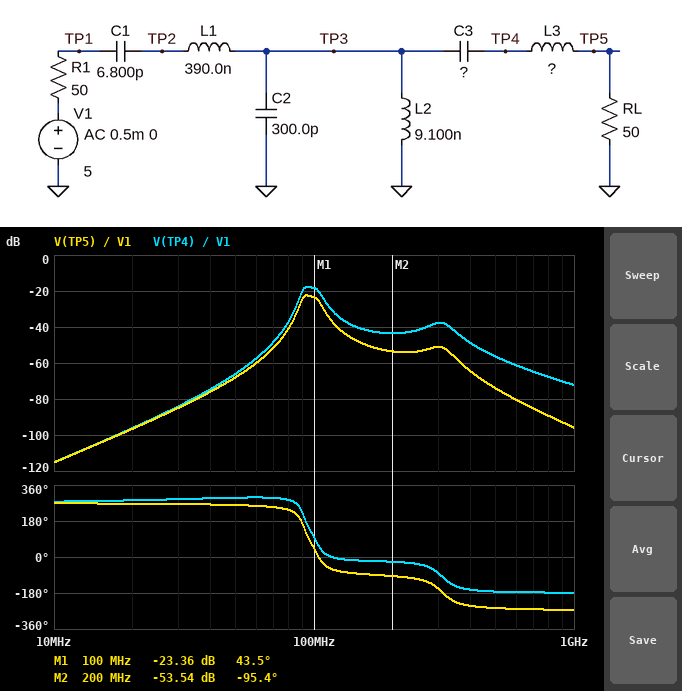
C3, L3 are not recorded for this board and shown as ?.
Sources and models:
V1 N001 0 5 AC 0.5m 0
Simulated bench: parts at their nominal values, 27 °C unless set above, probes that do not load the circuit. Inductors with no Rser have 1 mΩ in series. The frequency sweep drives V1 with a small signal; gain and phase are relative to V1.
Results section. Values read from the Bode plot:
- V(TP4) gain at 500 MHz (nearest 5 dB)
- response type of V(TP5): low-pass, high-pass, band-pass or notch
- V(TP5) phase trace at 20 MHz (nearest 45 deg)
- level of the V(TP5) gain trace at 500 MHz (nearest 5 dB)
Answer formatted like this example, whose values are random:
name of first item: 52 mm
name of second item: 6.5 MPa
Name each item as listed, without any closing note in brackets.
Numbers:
V(TP4) gain at 500 MHz: -55 dB
response type of V(TP5): low-pass, high-pass, band-pass or notch: band-pass
V(TP5) phase trace at 20 MHz: 270 deg
level of the V(TP5) gain trace at 500 MHz: -75 dB
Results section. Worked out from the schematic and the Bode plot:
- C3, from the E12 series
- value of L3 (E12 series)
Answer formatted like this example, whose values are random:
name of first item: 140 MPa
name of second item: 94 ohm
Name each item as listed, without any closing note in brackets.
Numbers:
C3, from the E12 series: 2.2 pF
value of L3: 120 nH
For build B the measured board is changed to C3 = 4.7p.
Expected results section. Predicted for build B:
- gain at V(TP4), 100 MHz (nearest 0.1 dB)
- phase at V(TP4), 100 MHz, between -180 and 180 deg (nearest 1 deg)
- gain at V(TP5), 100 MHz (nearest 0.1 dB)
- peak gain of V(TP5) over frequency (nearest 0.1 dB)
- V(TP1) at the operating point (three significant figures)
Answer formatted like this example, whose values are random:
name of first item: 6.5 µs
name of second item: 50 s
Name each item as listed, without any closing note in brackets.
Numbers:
gain at V(TP4), 100 MHz: -11.1 dB
phase at V(TP4), 100 MHz, between -180 and 180 deg: 90 deg
gain at V(TP5), 100 MHz: -16.3 dB
peak gain of V(TP5) over frequency: -15.0 dB
V(TP1) at the operating point: 5.00 V
